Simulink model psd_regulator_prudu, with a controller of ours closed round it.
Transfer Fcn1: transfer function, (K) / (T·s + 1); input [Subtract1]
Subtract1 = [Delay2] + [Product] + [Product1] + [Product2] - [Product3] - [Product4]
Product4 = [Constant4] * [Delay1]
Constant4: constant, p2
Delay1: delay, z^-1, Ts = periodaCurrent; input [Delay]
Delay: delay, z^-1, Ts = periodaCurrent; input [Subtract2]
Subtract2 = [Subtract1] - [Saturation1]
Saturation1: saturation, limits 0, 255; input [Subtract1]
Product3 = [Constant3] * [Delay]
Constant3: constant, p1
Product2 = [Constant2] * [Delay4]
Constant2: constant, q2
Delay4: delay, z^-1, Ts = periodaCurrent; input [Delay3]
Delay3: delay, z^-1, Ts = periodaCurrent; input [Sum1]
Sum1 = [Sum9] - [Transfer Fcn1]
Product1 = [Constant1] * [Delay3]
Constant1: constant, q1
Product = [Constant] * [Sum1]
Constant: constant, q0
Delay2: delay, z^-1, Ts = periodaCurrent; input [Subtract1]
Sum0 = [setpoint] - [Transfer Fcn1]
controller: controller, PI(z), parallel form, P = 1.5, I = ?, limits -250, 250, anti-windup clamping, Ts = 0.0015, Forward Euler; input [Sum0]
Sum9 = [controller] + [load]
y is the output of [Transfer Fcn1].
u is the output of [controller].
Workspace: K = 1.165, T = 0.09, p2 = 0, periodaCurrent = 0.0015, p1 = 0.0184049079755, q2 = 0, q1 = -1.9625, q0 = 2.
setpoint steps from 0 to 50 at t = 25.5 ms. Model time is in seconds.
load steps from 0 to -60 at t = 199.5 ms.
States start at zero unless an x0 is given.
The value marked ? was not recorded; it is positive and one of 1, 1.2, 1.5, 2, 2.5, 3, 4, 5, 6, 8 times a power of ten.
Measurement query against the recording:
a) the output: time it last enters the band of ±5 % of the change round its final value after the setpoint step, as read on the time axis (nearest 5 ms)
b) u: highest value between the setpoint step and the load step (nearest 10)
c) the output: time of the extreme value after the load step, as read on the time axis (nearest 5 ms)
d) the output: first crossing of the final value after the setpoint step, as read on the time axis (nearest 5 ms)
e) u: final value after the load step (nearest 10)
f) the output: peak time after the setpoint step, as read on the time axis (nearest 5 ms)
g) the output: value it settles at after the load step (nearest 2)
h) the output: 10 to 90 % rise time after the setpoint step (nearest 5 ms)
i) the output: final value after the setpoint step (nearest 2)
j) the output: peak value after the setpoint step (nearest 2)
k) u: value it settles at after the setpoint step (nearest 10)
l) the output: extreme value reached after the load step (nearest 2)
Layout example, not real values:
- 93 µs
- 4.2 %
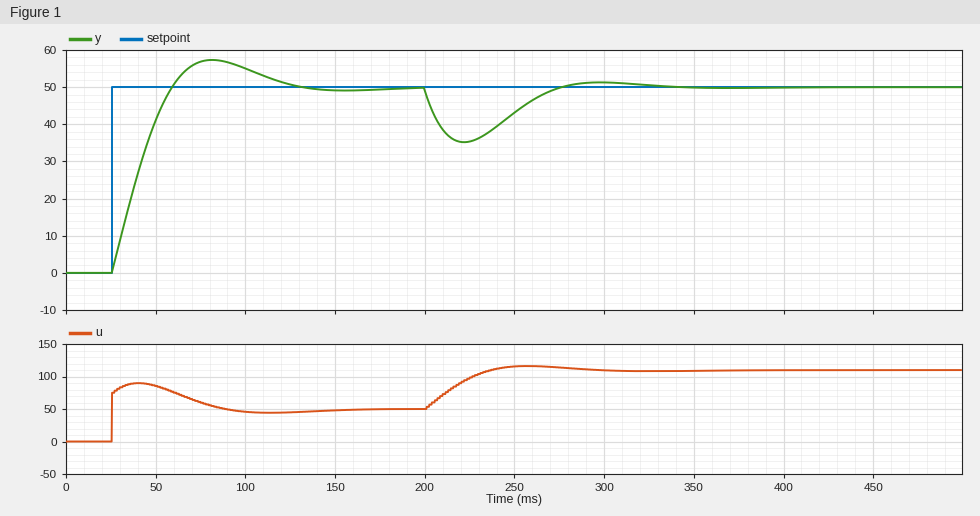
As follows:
- 115 ms
- 90
- 220 ms
- 60 ms
- 110
- 80 ms
- 50
- 25 ms
- 50
- 58
- 50
- 36
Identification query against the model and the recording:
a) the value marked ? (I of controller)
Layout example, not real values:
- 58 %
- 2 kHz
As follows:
- 100
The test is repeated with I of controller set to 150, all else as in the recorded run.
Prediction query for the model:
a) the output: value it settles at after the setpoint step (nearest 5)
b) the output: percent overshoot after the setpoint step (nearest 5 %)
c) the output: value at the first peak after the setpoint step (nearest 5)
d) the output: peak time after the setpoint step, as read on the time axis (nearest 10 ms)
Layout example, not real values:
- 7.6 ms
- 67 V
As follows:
- 50
- 25 %
- 60
- 70 ms
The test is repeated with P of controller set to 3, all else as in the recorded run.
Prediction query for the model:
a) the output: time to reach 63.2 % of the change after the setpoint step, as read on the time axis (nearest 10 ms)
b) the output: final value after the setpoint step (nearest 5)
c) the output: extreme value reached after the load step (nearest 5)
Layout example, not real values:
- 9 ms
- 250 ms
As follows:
- 40 ms
- 50
- 40
